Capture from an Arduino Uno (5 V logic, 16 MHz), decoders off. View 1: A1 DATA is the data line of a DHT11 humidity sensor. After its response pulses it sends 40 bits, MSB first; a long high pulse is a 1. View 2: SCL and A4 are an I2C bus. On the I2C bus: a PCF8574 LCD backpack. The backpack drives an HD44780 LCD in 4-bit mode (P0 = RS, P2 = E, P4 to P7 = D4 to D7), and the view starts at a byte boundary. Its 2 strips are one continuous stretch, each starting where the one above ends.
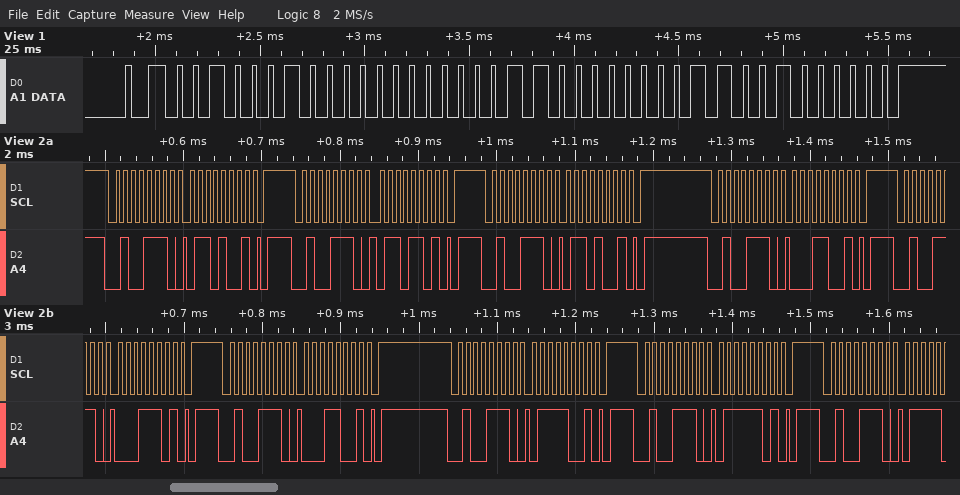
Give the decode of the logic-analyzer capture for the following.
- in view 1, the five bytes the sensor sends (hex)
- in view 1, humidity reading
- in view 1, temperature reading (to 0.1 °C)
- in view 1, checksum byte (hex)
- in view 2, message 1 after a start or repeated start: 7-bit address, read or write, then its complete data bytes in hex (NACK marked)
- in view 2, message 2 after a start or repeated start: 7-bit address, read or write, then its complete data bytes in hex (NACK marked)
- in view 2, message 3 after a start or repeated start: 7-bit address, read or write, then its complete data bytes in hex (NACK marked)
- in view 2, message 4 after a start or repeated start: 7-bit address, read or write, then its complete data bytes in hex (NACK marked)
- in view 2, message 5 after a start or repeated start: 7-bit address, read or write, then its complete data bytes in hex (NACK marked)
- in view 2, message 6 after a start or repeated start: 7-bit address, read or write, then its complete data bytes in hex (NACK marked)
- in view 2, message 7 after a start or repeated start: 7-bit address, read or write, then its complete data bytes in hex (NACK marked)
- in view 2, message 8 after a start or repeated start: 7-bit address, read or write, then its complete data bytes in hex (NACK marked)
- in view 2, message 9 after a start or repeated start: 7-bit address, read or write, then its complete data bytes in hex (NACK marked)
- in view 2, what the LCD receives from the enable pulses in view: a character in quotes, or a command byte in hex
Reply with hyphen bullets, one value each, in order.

- 22 00 18 06 40
- 34 %
- 24.6 °C
- 0x40
- 0x27 write: 69
- 0x27 write: 6D
- 0x27 write: 69
- 0x27 write: 19
- 0x27 write: 1D
- 0x27 write: 19
- 0x27 write: 79
- 0x27 write: 7D
- 0x27 write
- 'a'
